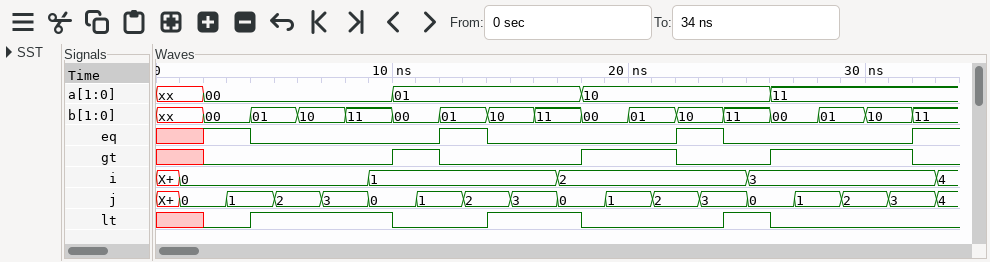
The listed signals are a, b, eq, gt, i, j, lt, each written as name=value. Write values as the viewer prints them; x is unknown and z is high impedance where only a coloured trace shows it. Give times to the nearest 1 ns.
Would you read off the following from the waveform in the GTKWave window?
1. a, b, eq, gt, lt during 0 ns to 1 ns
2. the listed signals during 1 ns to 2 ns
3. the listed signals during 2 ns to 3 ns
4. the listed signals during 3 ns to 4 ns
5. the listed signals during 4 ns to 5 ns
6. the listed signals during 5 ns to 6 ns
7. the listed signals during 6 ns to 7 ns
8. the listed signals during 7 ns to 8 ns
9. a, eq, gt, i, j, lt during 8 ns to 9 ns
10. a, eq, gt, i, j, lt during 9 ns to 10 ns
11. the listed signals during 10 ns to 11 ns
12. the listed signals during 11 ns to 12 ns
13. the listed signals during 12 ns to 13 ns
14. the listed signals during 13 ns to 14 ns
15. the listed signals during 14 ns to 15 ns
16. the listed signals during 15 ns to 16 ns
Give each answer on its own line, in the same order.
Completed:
a=xx, b=xx, eq=x, gt=x, lt=x
a=xx, b=xx, eq=x, gt=x, i=0, j=0, lt=x
a=00, b=00, eq=1, gt=0, i=0, j=0, lt=0
a=00, b=00, eq=1, gt=0, i=0, j=1, lt=0
a=00, b=01, eq=0, gt=0, i=0, j=1, lt=1
a=00, b=01, eq=0, gt=0, i=0, j=2, lt=1
a=00, b=10, eq=0, gt=0, i=0, j=2, lt=1
a=00, b=10, eq=0, gt=0, i=0, j=3, lt=1
a=00, eq=0, gt=0, i=0, j=3, lt=1
a=00, eq=0, gt=0, i=1, j=0, lt=1
a=01, b=00, eq=0, gt=1, i=1, j=0, lt=0
a=01, b=00, eq=0, gt=1, i=1, j=1, lt=0
a=01, b=01, eq=1, gt=0, i=1, j=1, lt=0
a=01, b=01, eq=1, gt=0, i=1, j=2, lt=0
a=01, b=10, eq=0, gt=0, i=1, j=2, lt=1
a=01, b=10, eq=0, gt=0, i=1, j=3, lt=1
